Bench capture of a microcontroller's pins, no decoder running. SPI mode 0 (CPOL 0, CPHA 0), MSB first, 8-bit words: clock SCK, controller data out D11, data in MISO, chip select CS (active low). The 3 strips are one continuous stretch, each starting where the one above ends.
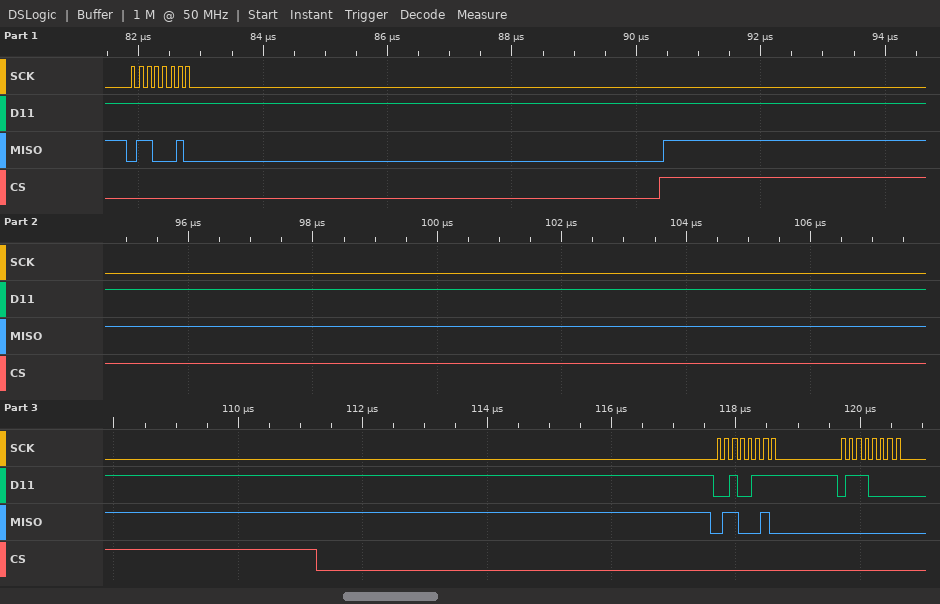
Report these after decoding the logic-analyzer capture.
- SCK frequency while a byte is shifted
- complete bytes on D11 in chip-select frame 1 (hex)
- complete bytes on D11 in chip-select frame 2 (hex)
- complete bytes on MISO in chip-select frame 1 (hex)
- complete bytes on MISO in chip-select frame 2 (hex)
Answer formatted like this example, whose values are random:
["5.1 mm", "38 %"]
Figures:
["8 MHz", "FF", "27 70", "62", "62 00"]
